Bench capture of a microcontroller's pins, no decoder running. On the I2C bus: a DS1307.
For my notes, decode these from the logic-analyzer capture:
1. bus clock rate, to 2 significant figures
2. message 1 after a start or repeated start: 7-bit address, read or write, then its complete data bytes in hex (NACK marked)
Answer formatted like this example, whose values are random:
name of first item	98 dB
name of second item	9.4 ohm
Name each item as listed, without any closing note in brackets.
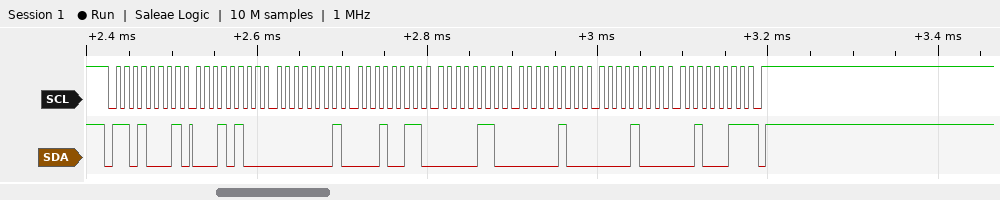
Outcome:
bus clock rate, to 2 significant figures	100 kHz
message 1 after a start or repeated start: 7-bit address, read or write, then its complete data bytes in hex	0x68 read: 14 01 13 06 04 08 23 NACK
